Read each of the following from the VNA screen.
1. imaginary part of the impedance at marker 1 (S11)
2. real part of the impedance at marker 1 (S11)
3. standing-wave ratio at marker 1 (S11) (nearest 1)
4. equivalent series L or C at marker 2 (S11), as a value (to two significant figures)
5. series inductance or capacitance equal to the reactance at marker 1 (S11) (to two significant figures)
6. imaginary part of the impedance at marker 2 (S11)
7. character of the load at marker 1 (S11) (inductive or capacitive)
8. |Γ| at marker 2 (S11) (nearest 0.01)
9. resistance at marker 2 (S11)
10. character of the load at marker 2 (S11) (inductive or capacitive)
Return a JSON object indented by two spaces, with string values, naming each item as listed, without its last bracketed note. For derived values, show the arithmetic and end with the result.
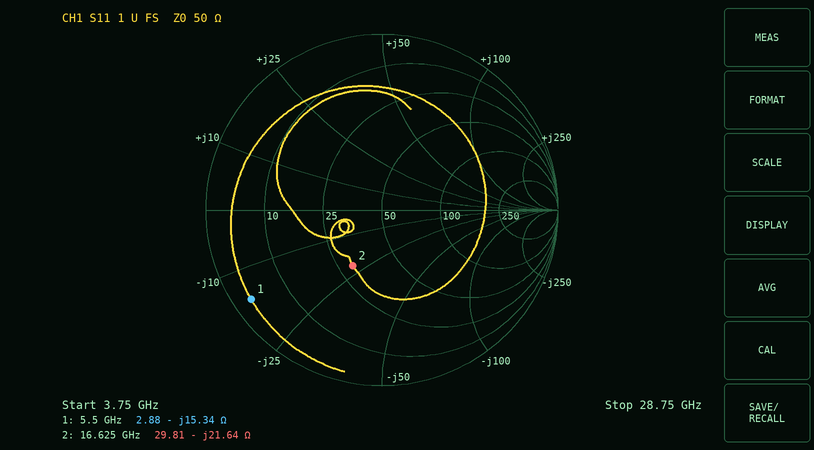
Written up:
{
  "imaginary part of the impedance at marker 1": "-15.34 Ω",
  "real part of the impedance at marker 1": "2.88 Ω",
  "standing-wave ratio at marker 1 (S11)": "19",
  "equivalent series L or C at marker 2 (S11), as a value": "C = 1/(2π × 16.625 GHz × 21.64 Ω) ≈ 442 fF, so 440 fF to two significant figures",
  "series inductance or capacitance equal to the reactance at marker 1 (S11)": "C = 1/(2π × 5.5 GHz × 15.34 Ω) ≈ 1.9 pF",
  "imaginary part of the impedance at marker 2": "-21.64 Ω",
  "character of the load at marker 1 (S11)": "capacitive",
  "|Γ| at marker 2 (S11)": "0.36",
  "resistance at marker 2": "29.81 Ω",
  "character of the load at marker 2 (S11)": "capacitive"
}
